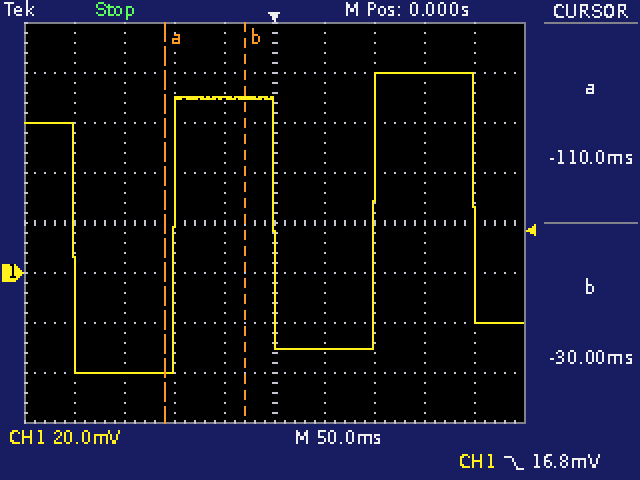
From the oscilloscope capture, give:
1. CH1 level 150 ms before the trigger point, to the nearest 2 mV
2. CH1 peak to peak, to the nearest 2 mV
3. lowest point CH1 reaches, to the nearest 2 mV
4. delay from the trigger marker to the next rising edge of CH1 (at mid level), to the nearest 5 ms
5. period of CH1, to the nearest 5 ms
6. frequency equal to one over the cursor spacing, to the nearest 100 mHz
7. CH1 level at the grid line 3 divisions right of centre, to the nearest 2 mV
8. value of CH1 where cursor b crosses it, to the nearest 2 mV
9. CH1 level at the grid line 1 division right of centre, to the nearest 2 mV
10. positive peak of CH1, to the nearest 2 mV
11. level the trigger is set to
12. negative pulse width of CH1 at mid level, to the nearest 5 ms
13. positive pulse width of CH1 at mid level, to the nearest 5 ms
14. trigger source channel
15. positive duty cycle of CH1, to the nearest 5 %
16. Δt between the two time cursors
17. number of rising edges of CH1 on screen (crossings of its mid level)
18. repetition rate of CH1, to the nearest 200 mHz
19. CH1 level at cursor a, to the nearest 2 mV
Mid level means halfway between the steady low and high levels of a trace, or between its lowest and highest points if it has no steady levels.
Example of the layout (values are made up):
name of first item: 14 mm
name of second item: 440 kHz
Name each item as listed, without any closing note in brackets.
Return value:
CH1 level 150 ms before the trigger point, to the nearest 2 mV: -40 mV
CH1 peak to peak, to the nearest 2 mV: 120 mV
lowest point CH1 reaches, to the nearest 2 mV: -40 mV
delay from the trigger marker to the next rising edge of CH1 (at mid level), to the nearest 5 ms: 100 ms
period of CH1, to the nearest 5 ms: 200 ms
frequency equal to one over the cursor spacing, to the nearest 100 mHz: 12.5 Hz
CH1 level at the grid line 3 divisions right of centre, to the nearest 2 mV: 80 mV
value of CH1 where cursor b crosses it, to the nearest 2 mV: 70 mV
CH1 level at the grid line 1 division right of centre, to the nearest 2 mV: -30 mV
positive peak of CH1, to the nearest 2 mV: 80 mV
level the trigger is set to: 16.8 mV
negative pulse width of CH1 at mid level, to the nearest 5 ms: 100 ms
positive pulse width of CH1 at mid level, to the nearest 5 ms: 100 ms
trigger source channel: CH1
positive duty cycle of CH1, to the nearest 5 %: 50 %
Δt between the two time cursors: 80 ms
number of rising edges of CH1 on screen: 2
repetition rate of CH1, to the nearest 200 mHz: 5.0 Hz
CH1 level at cursor a, to the nearest 2 mV: -40 mV
